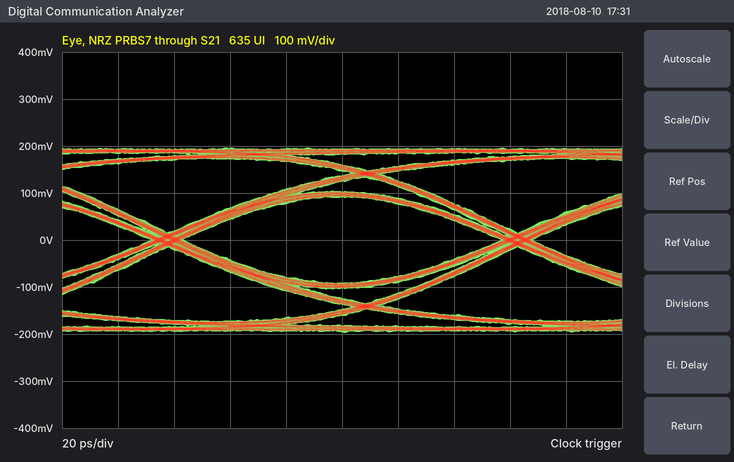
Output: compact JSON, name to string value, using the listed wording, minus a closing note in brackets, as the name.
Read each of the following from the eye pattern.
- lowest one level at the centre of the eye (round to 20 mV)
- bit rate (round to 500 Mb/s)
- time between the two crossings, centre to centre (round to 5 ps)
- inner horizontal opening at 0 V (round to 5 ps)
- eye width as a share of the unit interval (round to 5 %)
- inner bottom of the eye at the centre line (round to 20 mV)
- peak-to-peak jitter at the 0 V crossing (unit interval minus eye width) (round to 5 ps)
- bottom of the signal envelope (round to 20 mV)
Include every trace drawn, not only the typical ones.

{"lowest one level at the centre of the eye": "100 mV", "bit rate": "8.0 Gb/s", "time between the two crossings, centre to centre": "125 ps", "inner horizontal opening at 0 V": "115 ps", "eye width as a share of the unit interval": "90 %", "inner bottom of the eye at the centre line": "-100 mV", "peak-to-peak jitter at the 0 V crossing (unit interval minus eye width)": "10 ps", "bottom of the signal envelope": "-200 mV"}
